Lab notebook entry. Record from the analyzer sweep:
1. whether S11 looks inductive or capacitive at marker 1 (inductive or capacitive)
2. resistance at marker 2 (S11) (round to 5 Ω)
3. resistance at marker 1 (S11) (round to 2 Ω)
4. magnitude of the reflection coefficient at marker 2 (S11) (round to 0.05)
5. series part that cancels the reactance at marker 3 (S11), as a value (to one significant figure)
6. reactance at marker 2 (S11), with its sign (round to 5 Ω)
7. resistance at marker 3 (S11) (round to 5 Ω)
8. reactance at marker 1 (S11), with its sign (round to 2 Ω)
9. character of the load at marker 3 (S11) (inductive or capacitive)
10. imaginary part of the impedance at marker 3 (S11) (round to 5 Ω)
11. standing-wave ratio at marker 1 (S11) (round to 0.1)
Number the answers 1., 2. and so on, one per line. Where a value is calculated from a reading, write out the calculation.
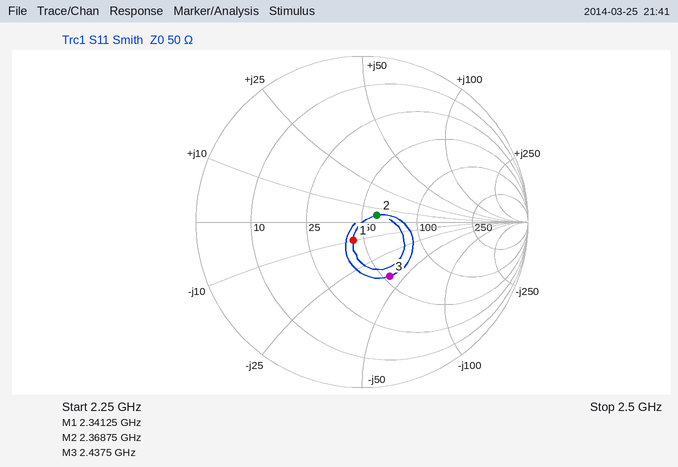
1. capacitive
2. 60 Ω
3. 44 Ω
4. 0.10
5. L = 40 Ω/(2π × 2.4375 GHz) ≈ 3 nH
6. +5 Ω
7. 55 Ω
8. -10 Ω
9. capacitive
10. -40 Ω
11. 1.3
